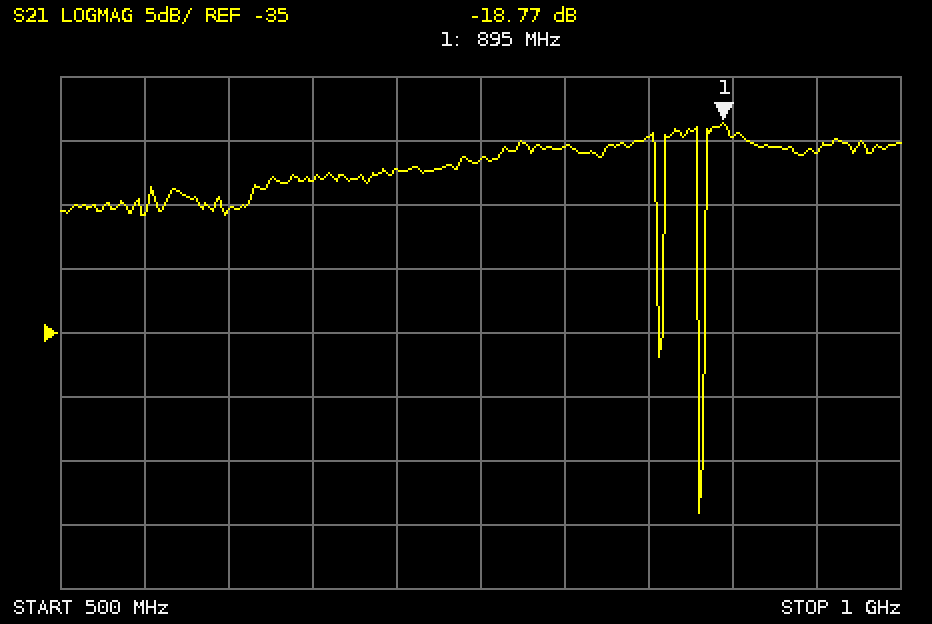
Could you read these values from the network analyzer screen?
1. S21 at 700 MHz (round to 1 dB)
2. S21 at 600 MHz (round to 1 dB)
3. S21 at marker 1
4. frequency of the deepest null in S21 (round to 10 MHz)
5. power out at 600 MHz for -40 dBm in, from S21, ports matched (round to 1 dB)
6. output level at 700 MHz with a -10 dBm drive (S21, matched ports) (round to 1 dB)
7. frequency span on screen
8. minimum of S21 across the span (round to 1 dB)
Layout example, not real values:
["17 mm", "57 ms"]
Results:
["-22 dB", "-25 dB", "-18.77 dB", "880 MHz", "-65 dBm", "-32 dBm", "500 MHz", "-49 dB"]
